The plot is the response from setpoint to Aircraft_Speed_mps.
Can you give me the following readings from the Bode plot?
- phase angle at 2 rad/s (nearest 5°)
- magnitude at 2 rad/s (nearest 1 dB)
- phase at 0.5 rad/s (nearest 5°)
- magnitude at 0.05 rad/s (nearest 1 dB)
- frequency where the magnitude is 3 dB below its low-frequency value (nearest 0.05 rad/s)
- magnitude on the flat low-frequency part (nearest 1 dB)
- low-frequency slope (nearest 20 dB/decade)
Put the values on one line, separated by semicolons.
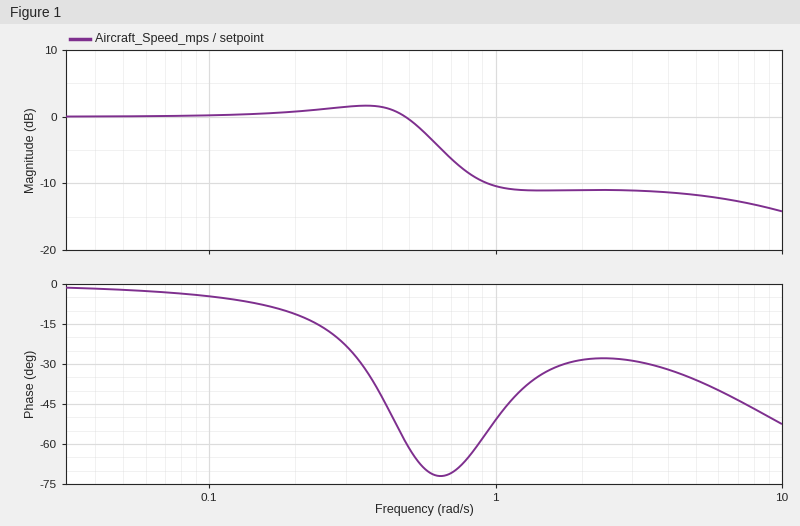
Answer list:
-30°; -11 dB; -60°; 0 dB; 0.60 rad/s; 0 dB; 0 dB/decade
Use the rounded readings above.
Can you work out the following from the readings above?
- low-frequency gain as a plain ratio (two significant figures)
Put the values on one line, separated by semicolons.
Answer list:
1.0
